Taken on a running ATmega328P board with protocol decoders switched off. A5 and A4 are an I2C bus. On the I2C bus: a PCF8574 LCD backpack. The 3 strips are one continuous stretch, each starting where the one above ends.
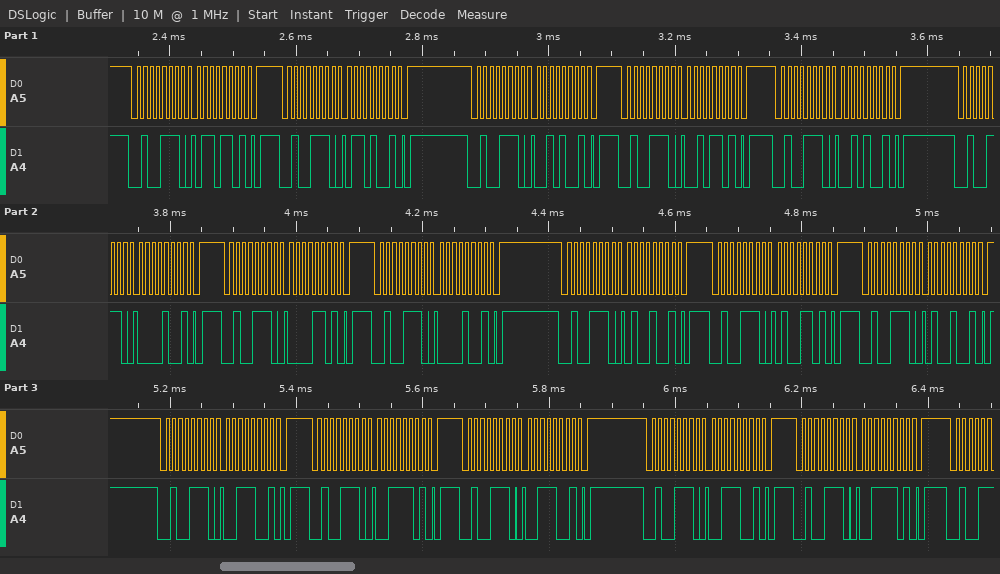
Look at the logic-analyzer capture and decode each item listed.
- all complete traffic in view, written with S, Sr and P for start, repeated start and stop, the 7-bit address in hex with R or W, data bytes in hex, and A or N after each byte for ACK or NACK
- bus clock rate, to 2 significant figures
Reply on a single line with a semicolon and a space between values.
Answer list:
S 27W A 6D A P S 27W A 69 A P S 27W A 29 A P S 27W A 2D A P S 27W A 29 A P S 27W A 09 A P S 27W A 0D A P S 27W A 09 A P S 27W A 49 A P S 27W A 4D A P S 27W A 49 A P S 27W A 39 A P S 27W A 3D A P S 27W A 39 A P S 27W A 39 A P S 27W A 3D A P; 100 kHz
